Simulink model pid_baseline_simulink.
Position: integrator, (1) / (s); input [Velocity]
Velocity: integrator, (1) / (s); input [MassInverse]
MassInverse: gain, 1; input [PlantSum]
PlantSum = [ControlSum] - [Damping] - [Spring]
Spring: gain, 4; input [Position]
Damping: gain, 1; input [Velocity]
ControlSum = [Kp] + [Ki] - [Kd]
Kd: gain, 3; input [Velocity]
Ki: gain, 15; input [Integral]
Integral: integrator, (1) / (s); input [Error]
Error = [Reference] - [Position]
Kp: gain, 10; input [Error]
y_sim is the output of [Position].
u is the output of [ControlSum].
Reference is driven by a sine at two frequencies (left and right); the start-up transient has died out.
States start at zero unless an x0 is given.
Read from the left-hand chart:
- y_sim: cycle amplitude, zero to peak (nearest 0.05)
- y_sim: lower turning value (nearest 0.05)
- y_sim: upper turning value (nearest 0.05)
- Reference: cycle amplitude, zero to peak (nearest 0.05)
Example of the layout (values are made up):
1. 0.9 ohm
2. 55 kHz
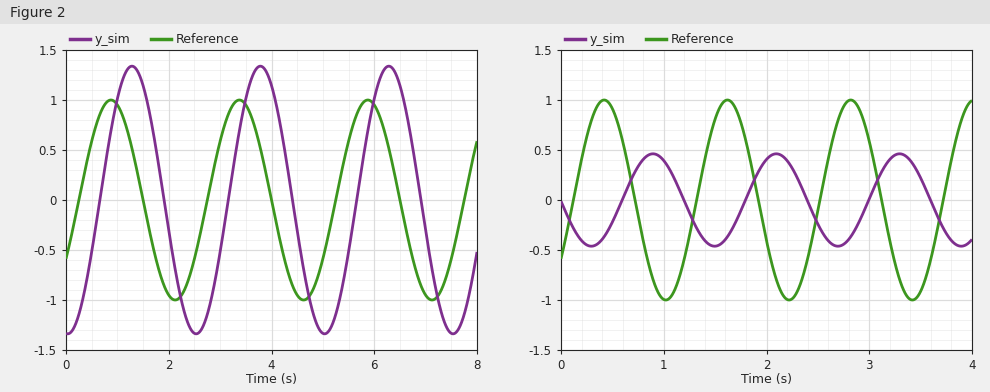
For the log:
1. 1.35
2. -1.35
3. 1.35
4. 1.00
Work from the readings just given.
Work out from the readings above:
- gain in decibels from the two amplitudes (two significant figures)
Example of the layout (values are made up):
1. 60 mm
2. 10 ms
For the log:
1. 2.6 dB
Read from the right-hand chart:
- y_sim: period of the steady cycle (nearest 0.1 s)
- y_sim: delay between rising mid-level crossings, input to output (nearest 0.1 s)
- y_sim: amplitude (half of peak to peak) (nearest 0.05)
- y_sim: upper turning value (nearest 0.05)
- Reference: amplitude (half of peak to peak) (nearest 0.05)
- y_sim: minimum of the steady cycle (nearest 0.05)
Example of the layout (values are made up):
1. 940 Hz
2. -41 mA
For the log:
1. 1.2 s
2. 0.5 s
3. 0.45
4. 0.45
5. 1.00
6. -0.45
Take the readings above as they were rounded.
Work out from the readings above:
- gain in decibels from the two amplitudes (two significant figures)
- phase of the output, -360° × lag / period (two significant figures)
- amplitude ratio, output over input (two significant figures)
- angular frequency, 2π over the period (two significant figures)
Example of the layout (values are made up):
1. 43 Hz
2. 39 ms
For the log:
1. -6.9 dB
2. -150°
3. 0.45
4. 5.2 rad/s
